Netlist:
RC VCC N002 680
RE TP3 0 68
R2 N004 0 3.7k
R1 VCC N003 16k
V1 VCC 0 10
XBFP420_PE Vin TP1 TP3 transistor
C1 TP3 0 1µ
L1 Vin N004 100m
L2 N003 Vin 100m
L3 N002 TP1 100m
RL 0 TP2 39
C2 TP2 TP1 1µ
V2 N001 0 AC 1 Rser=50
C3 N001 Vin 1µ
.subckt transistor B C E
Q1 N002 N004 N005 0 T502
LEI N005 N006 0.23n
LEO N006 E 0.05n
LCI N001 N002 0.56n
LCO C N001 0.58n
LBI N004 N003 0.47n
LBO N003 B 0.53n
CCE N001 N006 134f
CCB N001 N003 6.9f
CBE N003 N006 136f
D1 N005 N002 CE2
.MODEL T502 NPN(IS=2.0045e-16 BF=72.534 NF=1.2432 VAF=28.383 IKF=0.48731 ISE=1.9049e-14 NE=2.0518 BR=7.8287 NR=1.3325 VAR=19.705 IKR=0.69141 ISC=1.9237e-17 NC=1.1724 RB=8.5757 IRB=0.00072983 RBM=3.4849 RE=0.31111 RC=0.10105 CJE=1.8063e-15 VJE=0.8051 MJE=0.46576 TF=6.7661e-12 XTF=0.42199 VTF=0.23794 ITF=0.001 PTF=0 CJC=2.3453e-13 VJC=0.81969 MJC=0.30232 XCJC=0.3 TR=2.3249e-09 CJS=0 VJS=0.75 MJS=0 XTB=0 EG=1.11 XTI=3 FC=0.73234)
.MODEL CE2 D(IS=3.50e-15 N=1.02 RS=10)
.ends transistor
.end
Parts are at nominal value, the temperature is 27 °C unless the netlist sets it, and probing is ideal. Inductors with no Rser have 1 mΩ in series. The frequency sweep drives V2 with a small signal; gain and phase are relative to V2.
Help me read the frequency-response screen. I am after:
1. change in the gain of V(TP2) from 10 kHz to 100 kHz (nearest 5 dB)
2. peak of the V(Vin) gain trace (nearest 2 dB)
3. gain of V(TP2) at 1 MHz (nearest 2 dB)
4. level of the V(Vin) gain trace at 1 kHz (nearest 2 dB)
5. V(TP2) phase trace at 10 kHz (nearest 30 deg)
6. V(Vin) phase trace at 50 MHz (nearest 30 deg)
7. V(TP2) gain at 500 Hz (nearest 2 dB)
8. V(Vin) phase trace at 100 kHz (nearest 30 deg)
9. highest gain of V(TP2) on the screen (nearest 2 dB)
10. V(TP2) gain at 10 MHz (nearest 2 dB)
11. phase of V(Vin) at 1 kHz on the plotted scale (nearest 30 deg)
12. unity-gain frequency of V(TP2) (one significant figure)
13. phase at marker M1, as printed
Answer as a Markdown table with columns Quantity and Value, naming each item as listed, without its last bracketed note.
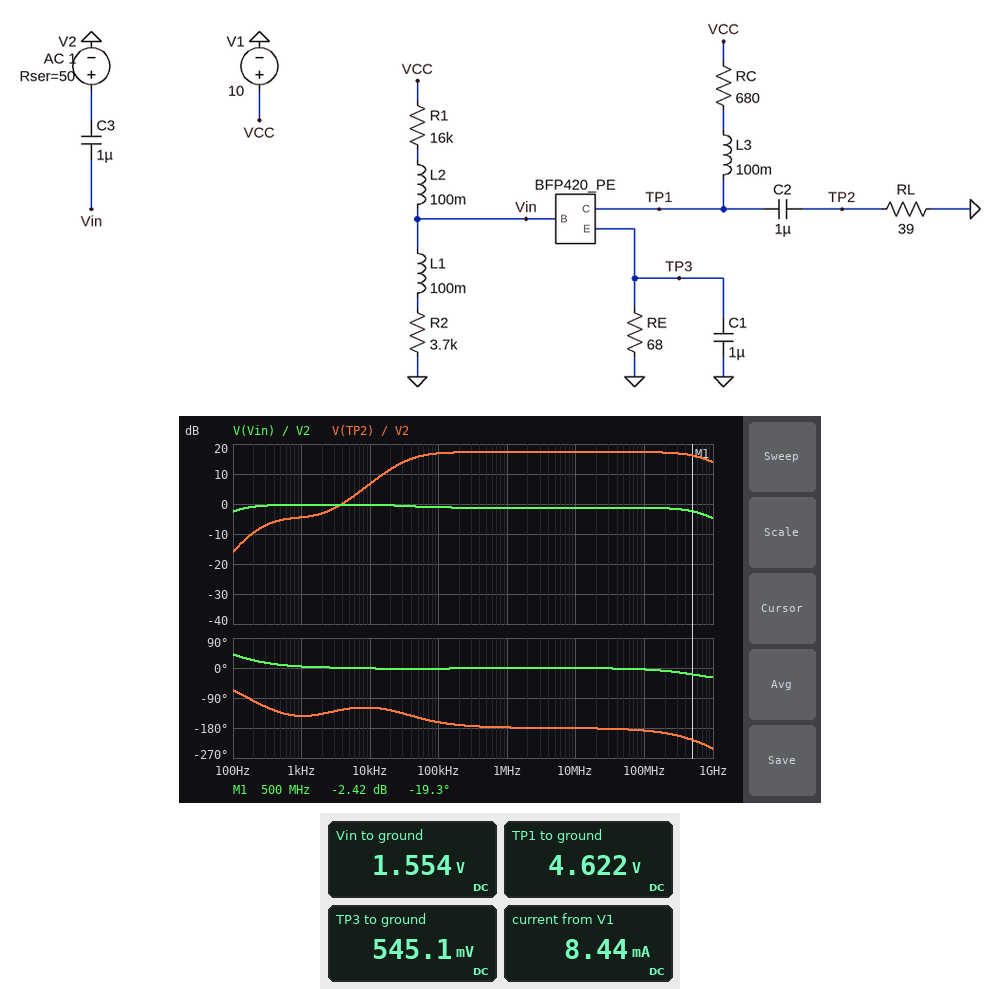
| Quantity | Value |
|---|---|
| change in the gain of V(TP2) from 10 kHz to 100 kHz | 10 dB |
| peak of the V(Vin) gain trace | 0 dB |
| gain of V(TP2) at 1 MHz | 18 dB |
| level of the V(Vin) gain trace at 1 kHz | 0 dB |
| V(TP2) phase trace at 10 kHz | -120 deg |
| V(Vin) phase trace at 50 MHz | 0 deg |
| V(TP2) gain at 500 Hz | -6 dB |
| V(Vin) phase trace at 100 kHz | 0 deg |
| highest gain of V(TP2) on the screen | 18 dB |
| V(TP2) gain at 10 MHz | 18 dB |
| phase of V(Vin) at 1 kHz on the plotted scale | 0 deg |
| unity-gain frequency of V(TP2) | 4 kHz |
| phase at marker M1, as printed | -19.3 deg |
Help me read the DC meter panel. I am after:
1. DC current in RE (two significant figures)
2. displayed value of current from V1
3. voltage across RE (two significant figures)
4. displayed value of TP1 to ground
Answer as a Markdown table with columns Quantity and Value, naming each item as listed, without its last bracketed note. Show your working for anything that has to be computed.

| Quantity | Value |
|---|---|
| DC current in RE | (545.1 mV) / 68 Ω = 8.0 mA |
| displayed value of current from V1 | 8.44 mA |
| voltage across RE | 545.1 mV = 550 mV |
| displayed value of TP1 to ground | 4.622 V |
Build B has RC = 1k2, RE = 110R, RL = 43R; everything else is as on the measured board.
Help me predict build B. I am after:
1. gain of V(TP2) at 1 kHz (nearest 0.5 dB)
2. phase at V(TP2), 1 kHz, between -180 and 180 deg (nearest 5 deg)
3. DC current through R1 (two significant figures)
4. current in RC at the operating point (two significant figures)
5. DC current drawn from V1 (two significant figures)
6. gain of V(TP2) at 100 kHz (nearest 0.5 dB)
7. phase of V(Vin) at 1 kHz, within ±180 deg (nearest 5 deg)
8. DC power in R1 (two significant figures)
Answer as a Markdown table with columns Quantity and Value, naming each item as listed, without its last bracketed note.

| Quantity | Value |
|---|---|
| gain of V(TP2) at 1 kHz | -7.0 dB |
| phase at V(TP2), 1 kHz, between -180 and 180 deg | -135 deg |
| DC current through R1 | 520 µA |
| current in RC at the operating point | 5.7 mA |
| DC current drawn from V1 | 6.2 mA |
| gain of V(TP2) at 100 kHz | 15.5 dB |
| phase of V(Vin) at 1 kHz, within ±180 deg | 5 deg |
| DC power in R1 | 4.4 mW |
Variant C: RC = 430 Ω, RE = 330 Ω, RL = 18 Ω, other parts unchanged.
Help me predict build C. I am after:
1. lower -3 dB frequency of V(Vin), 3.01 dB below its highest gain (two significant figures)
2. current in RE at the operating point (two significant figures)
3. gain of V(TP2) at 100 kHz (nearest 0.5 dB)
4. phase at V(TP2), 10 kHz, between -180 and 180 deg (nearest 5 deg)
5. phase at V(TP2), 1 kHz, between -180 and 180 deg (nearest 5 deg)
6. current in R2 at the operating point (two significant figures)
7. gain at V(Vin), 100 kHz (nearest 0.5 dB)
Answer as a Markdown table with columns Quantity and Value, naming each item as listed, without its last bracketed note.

| Quantity | Value |
|---|---|
| lower -3 dB frequency of V(Vin), 3.01 dB below its highest gain | 57 Hz |
| current in RE at the operating point | 2.5 mA |
| gain of V(TP2) at 100 kHz | 2.0 dB |
| phase at V(TP2), 10 kHz, between -180 and 180 deg | -130 deg |
| phase at V(TP2), 1 kHz, between -180 and 180 deg | -110 deg |
| current in R2 at the operating point | 480 µA |
| gain at V(Vin), 100 kHz | -0.5 dB |
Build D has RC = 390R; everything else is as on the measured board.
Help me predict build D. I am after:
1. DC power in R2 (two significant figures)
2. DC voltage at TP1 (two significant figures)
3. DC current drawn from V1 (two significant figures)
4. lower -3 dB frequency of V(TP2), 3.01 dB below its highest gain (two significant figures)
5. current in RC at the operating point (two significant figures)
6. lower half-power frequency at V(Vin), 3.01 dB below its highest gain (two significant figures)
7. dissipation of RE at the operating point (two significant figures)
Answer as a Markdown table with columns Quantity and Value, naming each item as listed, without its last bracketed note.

| Quantity | Value |
|---|---|
| DC power in R2 | 660 µW |
| DC voltage at TP1 | 6.8 V |
| DC current drawn from V1 | 8.7 mA |
| lower -3 dB frequency of V(TP2), 3.01 dB below its highest gain | 34 kHz |
| current in RC at the operating point | 8.1 mA |
| lower half-power frequency at V(Vin), 3.01 dB below its highest gain | 81 Hz |
| dissipation of RE at the operating point | 4.6 mW |
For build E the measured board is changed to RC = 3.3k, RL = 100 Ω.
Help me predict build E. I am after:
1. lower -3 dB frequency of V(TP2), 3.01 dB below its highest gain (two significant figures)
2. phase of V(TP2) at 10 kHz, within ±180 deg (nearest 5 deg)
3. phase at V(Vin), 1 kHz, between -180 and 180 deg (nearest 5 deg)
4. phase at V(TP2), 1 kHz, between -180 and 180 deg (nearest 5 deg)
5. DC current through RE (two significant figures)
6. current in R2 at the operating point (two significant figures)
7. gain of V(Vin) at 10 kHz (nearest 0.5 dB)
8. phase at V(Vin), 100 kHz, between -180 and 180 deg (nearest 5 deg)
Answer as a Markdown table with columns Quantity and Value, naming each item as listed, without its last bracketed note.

| Quantity | Value |
|---|---|
| lower -3 dB frequency of V(TP2), 3.01 dB below its highest gain | 9.3 kHz |
| phase of V(TP2) at 10 kHz, within ±180 deg | -135 deg |
| phase at V(Vin), 1 kHz, between -180 and 180 deg | 45 deg |
| phase at V(TP2), 1 kHz, between -180 and 180 deg | -70 deg |
| DC current through RE | 3.2 mA |
| current in R2 at the operating point | 320 µA |
| gain of V(Vin) at 10 kHz | -6.0 dB |
| phase at V(Vin), 100 kHz, between -180 and 180 deg | 0 deg |
